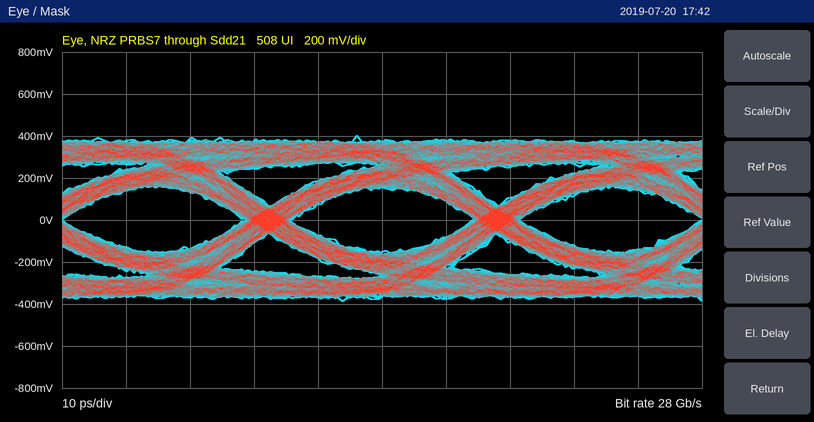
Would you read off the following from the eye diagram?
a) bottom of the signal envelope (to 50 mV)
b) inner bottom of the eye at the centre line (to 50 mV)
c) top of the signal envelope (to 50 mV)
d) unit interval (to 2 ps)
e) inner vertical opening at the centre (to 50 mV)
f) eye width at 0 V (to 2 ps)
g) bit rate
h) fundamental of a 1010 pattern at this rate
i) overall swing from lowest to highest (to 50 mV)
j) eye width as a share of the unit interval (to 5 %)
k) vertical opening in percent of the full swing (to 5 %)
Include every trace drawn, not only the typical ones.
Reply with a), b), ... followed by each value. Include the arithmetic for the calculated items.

a) -400 mV
b) -150 mV
c) 400 mV
d) 36 ps
e) 300 mV
f) 28 ps
g) 28 Gb/s
h) 14 GHz
i) 800 mV
j) 28 ps / 36 ps ≈ 77.8 %, so 80 % to the nearest 5 %
k) 300 mV / 800 mV ≈ 37.5 %, so 40 % to the nearest 5 %
